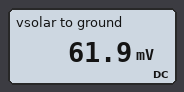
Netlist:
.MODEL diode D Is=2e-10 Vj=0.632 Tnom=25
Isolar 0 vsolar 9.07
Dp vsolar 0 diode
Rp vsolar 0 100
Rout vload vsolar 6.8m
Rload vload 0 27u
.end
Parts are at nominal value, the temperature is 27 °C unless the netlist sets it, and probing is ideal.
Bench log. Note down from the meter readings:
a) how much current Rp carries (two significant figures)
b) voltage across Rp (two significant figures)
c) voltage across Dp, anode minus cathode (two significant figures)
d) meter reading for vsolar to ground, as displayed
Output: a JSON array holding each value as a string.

["620 µA", "62 mV", "62 mV", "61.9 mV"]
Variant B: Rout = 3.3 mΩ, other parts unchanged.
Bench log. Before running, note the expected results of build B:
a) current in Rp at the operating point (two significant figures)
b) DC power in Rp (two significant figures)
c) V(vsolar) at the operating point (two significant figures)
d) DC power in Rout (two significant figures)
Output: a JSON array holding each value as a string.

["300 µA", "9.1 µW", "30 mV", "270 mW"]
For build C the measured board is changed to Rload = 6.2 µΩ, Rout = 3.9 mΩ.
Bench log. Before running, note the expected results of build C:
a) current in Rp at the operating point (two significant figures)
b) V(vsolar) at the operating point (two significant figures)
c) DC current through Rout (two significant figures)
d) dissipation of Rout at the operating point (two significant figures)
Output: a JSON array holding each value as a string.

["350 µA", "35 mV", "9.1 A", "320 mW"]
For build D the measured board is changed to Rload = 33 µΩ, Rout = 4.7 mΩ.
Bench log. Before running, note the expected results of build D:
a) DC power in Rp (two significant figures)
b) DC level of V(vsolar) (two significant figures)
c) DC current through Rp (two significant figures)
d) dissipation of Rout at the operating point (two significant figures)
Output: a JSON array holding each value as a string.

["18 µW", "43 mV", "430 µA", "390 mW"]
